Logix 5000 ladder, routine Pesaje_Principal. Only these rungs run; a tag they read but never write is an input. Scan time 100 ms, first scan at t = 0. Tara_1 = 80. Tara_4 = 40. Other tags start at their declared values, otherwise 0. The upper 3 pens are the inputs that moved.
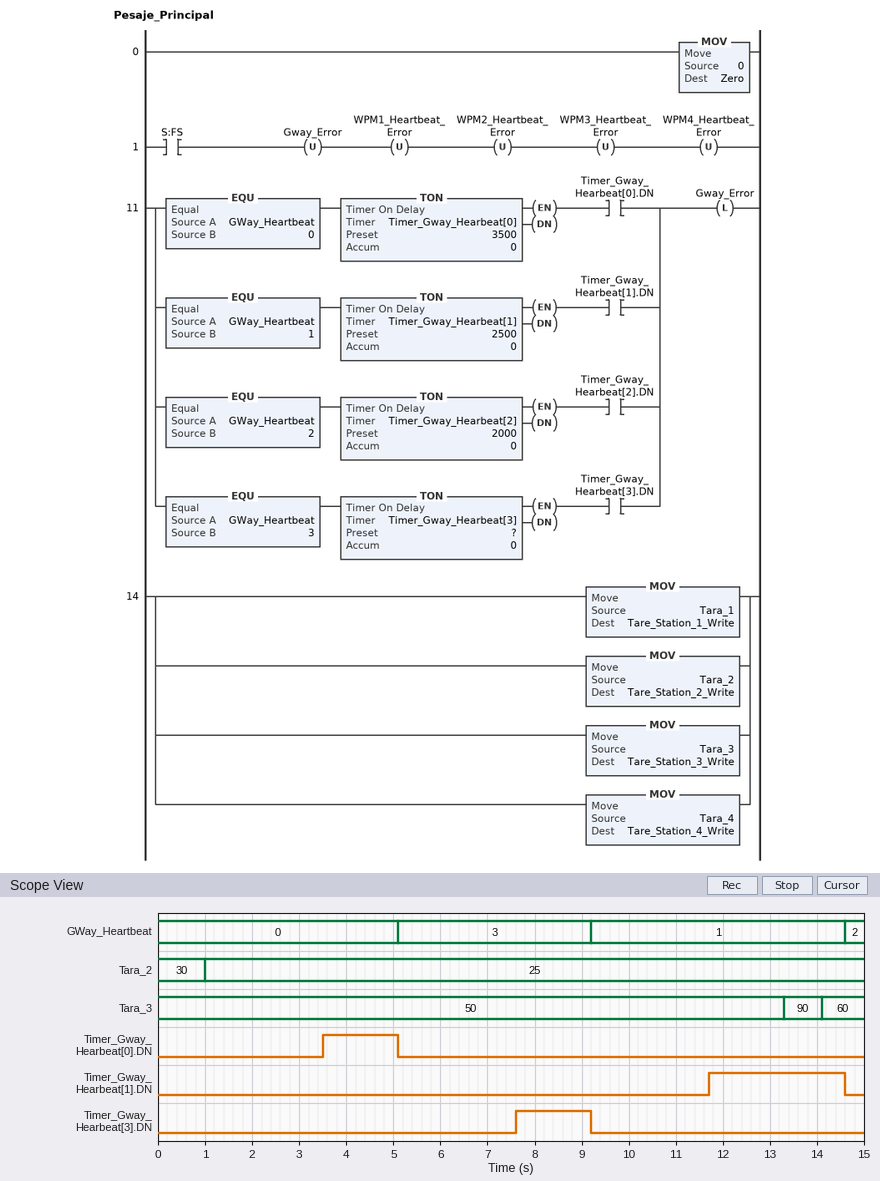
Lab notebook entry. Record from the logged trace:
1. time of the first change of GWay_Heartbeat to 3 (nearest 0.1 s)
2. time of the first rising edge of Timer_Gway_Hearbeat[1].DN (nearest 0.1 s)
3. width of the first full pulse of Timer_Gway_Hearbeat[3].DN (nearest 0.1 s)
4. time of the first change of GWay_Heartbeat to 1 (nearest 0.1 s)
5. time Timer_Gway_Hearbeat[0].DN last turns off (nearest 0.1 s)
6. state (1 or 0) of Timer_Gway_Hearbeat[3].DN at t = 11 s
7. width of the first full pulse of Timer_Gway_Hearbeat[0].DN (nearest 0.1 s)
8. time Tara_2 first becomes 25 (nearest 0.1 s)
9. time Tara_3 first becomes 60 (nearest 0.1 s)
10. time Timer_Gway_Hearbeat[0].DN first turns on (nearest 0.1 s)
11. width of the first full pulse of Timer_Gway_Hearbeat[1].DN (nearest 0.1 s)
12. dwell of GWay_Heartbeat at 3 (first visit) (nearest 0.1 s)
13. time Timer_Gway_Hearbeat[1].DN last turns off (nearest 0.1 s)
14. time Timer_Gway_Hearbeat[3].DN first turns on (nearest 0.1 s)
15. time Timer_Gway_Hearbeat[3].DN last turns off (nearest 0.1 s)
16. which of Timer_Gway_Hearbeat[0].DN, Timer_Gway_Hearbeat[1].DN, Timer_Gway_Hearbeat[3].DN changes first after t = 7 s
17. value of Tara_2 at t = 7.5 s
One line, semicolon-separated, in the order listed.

5.1 s; 11.7 s; 1.6 s; 9.2 s; 5.1 s; 0; 1.6 s; 1.0 s; 14.1 s; 3.5 s; 2.9 s; 4.1 s; 14.6 s; 7.6 s; 9.2 s; Timer_Gway_Hearbeat[3].DN; 25
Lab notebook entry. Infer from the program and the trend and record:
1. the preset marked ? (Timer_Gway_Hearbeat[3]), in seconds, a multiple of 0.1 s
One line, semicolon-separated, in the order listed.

2.5 s
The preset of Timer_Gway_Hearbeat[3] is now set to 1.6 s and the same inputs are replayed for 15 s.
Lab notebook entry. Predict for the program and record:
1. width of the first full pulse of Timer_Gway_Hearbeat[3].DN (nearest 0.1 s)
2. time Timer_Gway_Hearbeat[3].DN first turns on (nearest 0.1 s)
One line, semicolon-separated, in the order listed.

2.5 s; 6.7 s
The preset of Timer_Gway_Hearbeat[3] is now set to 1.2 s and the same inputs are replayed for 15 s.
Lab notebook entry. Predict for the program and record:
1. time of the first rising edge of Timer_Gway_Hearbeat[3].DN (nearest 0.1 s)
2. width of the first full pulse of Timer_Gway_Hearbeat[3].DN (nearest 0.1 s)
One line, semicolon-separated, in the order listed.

6.3 s; 2.9 s
